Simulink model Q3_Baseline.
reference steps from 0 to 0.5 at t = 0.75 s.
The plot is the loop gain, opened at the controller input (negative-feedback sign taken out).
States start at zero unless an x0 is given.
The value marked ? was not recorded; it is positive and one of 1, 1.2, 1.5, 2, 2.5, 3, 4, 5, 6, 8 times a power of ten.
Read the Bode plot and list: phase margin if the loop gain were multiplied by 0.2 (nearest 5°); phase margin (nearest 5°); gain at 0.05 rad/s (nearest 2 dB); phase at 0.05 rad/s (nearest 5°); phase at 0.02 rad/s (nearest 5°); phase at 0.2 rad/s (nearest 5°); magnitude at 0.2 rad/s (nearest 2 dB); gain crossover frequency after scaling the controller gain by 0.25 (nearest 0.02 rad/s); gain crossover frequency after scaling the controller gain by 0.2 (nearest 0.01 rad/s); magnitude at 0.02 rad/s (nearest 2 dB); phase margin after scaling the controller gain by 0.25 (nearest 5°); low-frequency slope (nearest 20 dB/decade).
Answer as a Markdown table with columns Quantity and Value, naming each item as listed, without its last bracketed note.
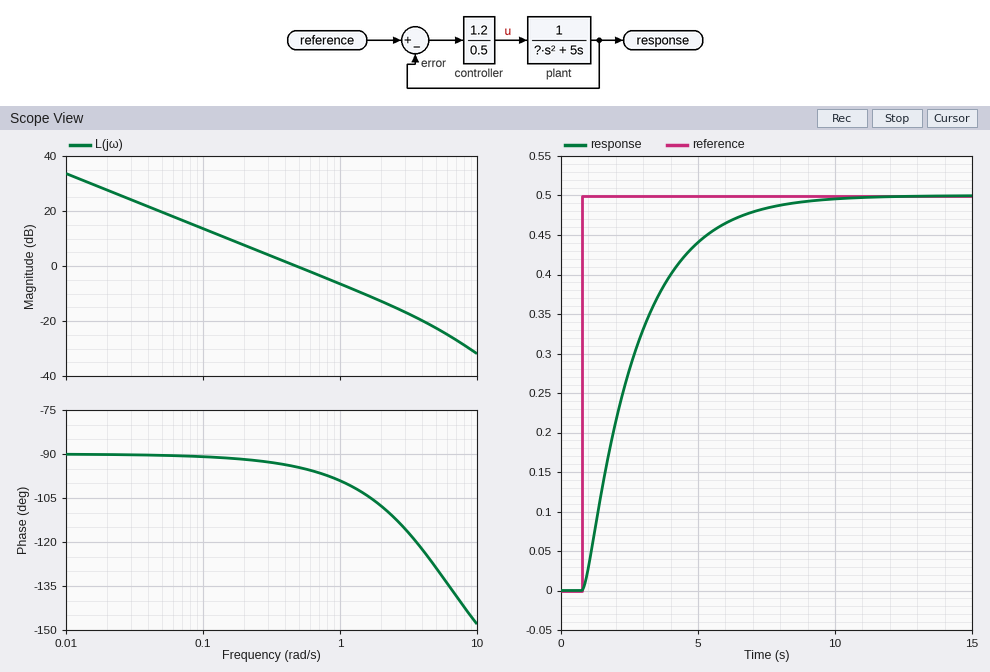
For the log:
| Quantity | Value |
|---|---|
| phase margin if the loop gain were multiplied by 0.2 | 90° |
| phase margin | 85° |
| gain at 0.05 rad/s | 20 dB |
| phase at 0.05 rad/s | -90° |
| phase at 0.02 rad/s | -90° |
| phase at 0.2 rad/s | -90° |
| magnitude at 0.2 rad/s | 8 dB |
| gain crossover frequency after scaling the controller gain by 0.25 | 0.12 rad/s |
| gain crossover frequency after scaling the controller gain by 0.2 | 0.10 rad/s |
| magnitude at 0.02 rad/s | 28 dB |
| phase margin after scaling the controller gain by 0.25 | 90° |
| low-frequency slope | -20 dB/decade |
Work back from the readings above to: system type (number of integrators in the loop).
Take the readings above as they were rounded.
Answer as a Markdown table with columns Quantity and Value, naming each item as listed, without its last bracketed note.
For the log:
| Quantity | Value |
|---|---|
| system type | 1 |
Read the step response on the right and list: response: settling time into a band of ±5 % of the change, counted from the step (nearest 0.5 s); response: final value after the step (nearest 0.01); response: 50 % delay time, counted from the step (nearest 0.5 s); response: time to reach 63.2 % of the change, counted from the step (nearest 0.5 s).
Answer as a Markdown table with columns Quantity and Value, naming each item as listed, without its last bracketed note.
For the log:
| Quantity | Value |
|---|---|
| response: settling time into a band of ±5 % of the change, counted from the step | 6.0 s |
| response: final value after the step | 0.50 |
| response: 50 % delay time, counted from the step | 1.5 s |
| response: time to reach 63.2 % of the change, counted from the step | 2.0 s |
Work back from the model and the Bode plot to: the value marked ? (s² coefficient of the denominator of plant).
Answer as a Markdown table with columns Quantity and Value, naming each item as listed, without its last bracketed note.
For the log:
| Quantity | Value |
|---|---|
| the value marked ? | 0.8 |
